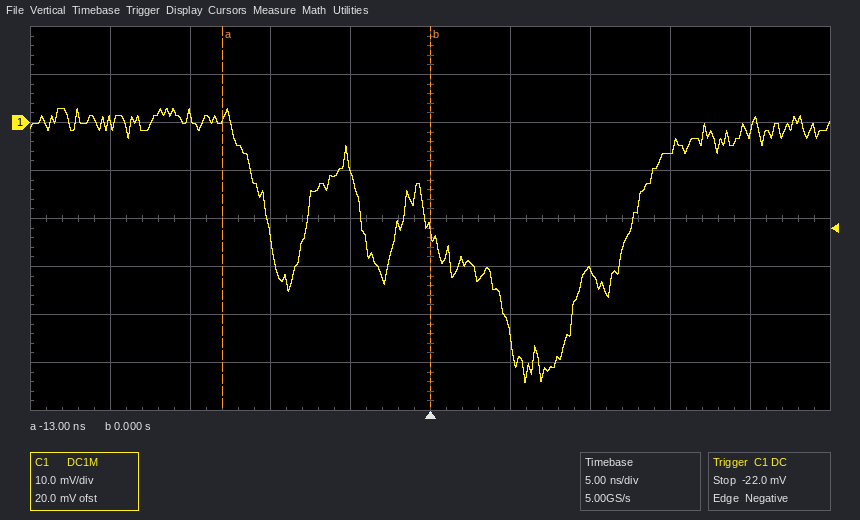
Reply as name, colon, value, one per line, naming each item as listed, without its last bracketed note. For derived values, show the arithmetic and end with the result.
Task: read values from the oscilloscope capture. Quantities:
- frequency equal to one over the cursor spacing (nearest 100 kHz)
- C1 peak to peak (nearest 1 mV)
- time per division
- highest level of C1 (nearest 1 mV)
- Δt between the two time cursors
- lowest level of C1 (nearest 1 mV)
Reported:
frequency equal to one over the cursor spacing: 1 / 13.0 ns ≈ 76.9 MHz
C1 peak to peak: 3 mV − (-54 mV) = 57 mV
time per division: 5 ns
highest level of C1: 3 mV
Δt between the two time cursors: 0 s − (-13 ns) = 13.0 ns
lowest level of C1: -54 mV
